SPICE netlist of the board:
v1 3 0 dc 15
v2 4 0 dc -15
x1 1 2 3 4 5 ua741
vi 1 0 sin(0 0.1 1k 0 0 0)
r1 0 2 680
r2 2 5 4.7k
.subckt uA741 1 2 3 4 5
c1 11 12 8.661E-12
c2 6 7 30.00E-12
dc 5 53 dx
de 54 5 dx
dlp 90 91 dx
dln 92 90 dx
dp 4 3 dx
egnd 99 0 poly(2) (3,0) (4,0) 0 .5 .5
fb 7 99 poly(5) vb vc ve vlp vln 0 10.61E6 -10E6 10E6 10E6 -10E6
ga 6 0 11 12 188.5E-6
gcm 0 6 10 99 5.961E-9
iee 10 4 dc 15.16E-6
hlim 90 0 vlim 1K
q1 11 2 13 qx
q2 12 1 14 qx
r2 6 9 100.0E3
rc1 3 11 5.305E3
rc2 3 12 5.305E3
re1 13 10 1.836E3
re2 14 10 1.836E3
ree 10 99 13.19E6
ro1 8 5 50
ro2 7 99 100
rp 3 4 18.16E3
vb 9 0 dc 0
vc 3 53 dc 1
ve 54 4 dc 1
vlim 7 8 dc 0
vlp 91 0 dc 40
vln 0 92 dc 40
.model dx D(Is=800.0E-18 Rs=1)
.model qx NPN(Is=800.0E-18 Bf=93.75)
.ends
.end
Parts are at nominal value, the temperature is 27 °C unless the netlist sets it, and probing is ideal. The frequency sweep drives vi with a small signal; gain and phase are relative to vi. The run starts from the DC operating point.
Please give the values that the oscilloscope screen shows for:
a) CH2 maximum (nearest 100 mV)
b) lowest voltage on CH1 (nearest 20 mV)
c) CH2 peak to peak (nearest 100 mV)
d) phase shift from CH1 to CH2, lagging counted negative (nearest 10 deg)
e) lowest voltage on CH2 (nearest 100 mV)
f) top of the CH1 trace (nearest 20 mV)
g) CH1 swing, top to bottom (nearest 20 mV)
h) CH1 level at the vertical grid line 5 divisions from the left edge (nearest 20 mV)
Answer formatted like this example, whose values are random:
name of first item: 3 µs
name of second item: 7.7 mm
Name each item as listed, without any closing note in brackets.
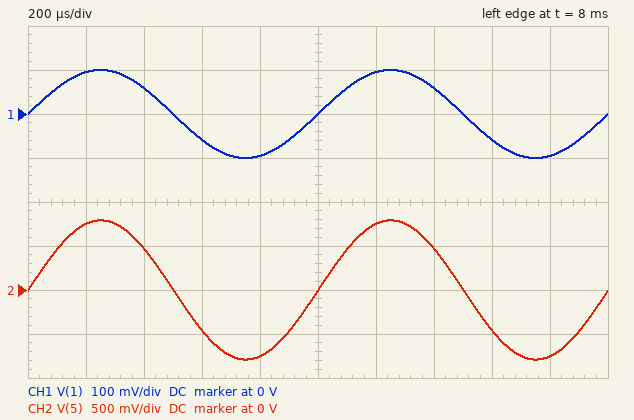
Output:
CH2 maximum: 800 mV
lowest voltage on CH1: -100 mV
CH2 peak to peak: 1.6 V
phase shift from CH1 to CH2, lagging counted negative: 0 deg
lowest voltage on CH2: -800 mV
top of the CH1 trace: 100 mV
CH1 swing, top to bottom: 200 mV
CH1 level at the vertical grid line 5 divisions from the left edge: 0 V
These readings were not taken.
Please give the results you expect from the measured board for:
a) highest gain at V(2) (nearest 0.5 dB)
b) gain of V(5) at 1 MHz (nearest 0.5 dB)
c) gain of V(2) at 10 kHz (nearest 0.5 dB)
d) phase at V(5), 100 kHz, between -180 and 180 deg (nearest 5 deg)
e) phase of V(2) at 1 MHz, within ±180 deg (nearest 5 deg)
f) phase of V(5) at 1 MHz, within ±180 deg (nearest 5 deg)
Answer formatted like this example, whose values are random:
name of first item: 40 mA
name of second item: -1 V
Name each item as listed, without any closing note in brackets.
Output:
highest gain at V(2): 0 dB
gain of V(5) at 1 MHz: -1.0 dB
gain of V(2) at 10 kHz: 0 dB
phase at V(5), 100 kHz, between -180 and 180 deg: -40 deg
phase of V(2) at 1 MHz, within ±180 deg: -115 deg
phase of V(5) at 1 MHz, within ±180 deg: -115 deg
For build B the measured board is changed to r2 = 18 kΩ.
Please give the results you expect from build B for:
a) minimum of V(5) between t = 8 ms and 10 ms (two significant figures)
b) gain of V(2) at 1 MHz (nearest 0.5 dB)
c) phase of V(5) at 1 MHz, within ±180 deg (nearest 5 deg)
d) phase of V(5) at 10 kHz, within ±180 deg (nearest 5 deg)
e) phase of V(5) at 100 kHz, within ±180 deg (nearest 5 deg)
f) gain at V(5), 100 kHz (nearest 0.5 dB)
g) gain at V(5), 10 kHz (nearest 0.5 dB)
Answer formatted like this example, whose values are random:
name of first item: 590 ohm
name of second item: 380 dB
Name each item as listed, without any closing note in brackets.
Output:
minimum of V(5) between t = 8 ms and 10 ms: -2.7 V
gain of V(2) at 1 MHz: -30.0 dB
phase of V(5) at 1 MHz, within ±180 deg: -120 deg
phase of V(5) at 10 kHz, within ±180 deg: -15 deg
phase of V(5) at 100 kHz, within ±180 deg: -75 deg
gain at V(5), 100 kHz: 19.5 dB
gain at V(5), 10 kHz: 28.5 dB
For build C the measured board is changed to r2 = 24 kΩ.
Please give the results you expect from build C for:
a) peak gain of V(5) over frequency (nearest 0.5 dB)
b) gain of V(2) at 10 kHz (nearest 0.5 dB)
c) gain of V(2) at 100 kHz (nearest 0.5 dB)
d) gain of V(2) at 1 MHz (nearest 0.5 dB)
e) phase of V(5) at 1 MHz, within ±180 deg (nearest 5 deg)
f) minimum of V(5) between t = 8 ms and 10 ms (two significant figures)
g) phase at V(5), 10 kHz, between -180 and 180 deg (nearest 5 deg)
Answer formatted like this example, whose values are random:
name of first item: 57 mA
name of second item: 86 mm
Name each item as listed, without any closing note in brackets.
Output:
peak gain of V(5) over frequency: 31.0 dB
gain of V(2) at 10 kHz: -0.5 dB
gain of V(2) at 100 kHz: -11.5 dB
gain of V(2) at 1 MHz: -32.5 dB
phase of V(5) at 1 MHz, within ±180 deg: -120 deg
minimum of V(5) between t = 8 ms and 10 ms: -3.6 V
phase at V(5), 10 kHz, between -180 and 180 deg: -20 deg
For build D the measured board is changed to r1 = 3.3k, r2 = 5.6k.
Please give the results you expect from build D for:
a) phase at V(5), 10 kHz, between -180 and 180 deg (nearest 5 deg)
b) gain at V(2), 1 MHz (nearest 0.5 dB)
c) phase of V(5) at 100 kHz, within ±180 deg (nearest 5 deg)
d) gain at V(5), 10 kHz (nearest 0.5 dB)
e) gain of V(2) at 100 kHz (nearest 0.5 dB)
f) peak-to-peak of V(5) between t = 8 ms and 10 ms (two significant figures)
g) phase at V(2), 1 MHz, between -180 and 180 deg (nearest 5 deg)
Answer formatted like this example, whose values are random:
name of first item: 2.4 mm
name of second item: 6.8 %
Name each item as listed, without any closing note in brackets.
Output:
phase at V(5), 10 kHz, between -180 and 180 deg: 0 deg
gain at V(2), 1 MHz: -9.0 dB
phase of V(5) at 100 kHz, within ±180 deg: -15 deg
gain at V(5), 10 kHz: 8.5 dB
gain of V(2) at 100 kHz: 0 dB
peak-to-peak of V(5) between t = 8 ms and 10 ms: 540 mV
phase at V(2), 1 MHz, between -180 and 180 deg: -100 deg
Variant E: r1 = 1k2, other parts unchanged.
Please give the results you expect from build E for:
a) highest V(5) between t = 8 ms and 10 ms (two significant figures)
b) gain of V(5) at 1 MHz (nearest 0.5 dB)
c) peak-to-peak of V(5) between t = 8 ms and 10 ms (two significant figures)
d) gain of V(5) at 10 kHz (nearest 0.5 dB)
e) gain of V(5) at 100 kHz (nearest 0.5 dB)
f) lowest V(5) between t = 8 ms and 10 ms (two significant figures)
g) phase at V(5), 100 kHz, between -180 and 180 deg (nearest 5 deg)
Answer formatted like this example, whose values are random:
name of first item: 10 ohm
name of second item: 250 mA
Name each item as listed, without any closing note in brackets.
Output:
highest V(5) between t = 8 ms and 10 ms: 490 mV
gain of V(5) at 1 MHz: -0.5 dB
peak-to-peak of V(5) between t = 8 ms and 10 ms: 980 mV
gain of V(5) at 10 kHz: 14.0 dB
gain of V(5) at 100 kHz: 13.0 dB
lowest V(5) between t = 8 ms and 10 ms: -490 mV
phase at V(5), 100 kHz, between -180 and 180 deg: -25 deg
